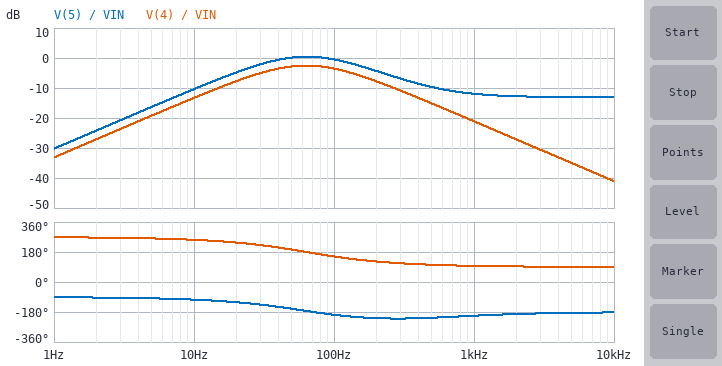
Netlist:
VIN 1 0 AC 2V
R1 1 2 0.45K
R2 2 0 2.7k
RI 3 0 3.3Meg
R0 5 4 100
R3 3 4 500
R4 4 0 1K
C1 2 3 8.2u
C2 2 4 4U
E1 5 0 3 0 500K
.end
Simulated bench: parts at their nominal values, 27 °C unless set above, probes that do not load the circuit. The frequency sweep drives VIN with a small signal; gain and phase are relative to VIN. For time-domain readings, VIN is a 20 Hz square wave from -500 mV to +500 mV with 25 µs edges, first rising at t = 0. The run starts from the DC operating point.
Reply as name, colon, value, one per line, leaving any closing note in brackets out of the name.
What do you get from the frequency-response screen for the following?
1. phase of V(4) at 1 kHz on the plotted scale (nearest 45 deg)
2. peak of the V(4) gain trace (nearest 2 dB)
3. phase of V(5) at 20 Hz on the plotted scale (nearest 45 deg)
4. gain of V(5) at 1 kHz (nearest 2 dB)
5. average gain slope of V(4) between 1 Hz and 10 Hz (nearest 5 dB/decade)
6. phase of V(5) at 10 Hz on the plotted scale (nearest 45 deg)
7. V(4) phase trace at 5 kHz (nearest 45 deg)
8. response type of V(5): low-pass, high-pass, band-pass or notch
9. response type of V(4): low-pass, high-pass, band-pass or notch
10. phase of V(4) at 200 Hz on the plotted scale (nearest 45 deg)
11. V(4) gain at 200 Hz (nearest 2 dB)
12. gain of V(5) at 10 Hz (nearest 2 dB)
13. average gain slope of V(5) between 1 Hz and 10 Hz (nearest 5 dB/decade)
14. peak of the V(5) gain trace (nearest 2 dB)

phase of V(4) at 1 kHz on the plotted scale: 90 deg
peak of the V(4) gain trace: -2 dB
phase of V(5) at 20 Hz on the plotted scale: -135 deg
gain of V(5) at 1 kHz: -12 dB
average gain slope of V(4) between 1 Hz and 10 Hz: 20 dB/decade
phase of V(5) at 10 Hz on the plotted scale: -90 deg
V(4) phase trace at 5 kHz: 90 deg
response type of V(5): low-pass, high-pass, band-pass or notch: band-pass
response type of V(4): low-pass, high-pass, band-pass or notch: band-pass
phase of V(4) at 200 Hz on the plotted scale: 135 deg
V(4) gain at 200 Hz: -8 dB
gain of V(5) at 10 Hz: -10 dB
average gain slope of V(5) between 1 Hz and 10 Hz: 20 dB/decade
peak of the V(5) gain trace: 0 dB
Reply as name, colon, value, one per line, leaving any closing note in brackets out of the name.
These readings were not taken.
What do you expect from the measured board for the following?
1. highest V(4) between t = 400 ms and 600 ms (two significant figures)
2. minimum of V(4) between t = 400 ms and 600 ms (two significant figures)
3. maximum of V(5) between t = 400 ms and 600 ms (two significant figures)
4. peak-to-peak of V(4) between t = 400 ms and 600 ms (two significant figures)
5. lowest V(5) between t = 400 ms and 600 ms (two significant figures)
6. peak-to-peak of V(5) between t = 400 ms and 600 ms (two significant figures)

highest V(4) between t = 400 ms and 600 ms: 540 mV
minimum of V(4) between t = 400 ms and 600 ms: -540 mV
maximum of V(5) between t = 400 ms and 600 ms: 760 mV
peak-to-peak of V(4) between t = 400 ms and 600 ms: 1.1 V
lowest V(5) between t = 400 ms and 600 ms: -760 mV
peak-to-peak of V(5) between t = 400 ms and 600 ms: 1.5 V
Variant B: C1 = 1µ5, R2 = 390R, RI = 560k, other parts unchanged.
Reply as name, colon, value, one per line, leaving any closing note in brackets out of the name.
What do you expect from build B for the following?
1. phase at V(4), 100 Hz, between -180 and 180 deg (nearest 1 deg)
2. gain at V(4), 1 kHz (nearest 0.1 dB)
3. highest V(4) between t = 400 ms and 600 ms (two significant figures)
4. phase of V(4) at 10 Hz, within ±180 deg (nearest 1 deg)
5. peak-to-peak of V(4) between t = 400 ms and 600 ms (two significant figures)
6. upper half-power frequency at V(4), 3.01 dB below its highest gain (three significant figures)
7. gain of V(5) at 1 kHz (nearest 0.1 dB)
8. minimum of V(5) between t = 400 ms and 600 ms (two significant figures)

phase at V(4), 100 Hz, between -180 and 180 deg: -134 deg
gain at V(4), 1 kHz: -21.1 dB
highest V(4) between t = 400 ms and 600 ms: 200 mV
phase of V(4) at 10 Hz, within ±180 deg: -94 deg
peak-to-peak of V(4) between t = 400 ms and 600 ms: 400 mV
upper half-power frequency at V(4), 3.01 dB below its highest gain: 394 Hz
gain of V(5) at 1 kHz: -11.2 dB
minimum of V(5) between t = 400 ms and 600 ms: -380 mV
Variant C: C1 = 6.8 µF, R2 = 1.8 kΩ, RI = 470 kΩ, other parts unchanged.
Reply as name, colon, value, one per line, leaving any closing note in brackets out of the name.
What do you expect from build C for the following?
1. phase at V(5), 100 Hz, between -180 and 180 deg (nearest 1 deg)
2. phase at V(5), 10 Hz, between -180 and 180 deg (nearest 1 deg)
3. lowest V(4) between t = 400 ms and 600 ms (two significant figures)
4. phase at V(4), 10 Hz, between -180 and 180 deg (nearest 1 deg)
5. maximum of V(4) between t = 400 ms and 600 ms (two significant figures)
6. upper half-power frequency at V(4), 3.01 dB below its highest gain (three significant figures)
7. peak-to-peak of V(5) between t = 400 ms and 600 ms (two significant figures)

phase at V(5), 100 Hz, between -180 and 180 deg: 169 deg
phase at V(5), 10 Hz, between -180 and 180 deg: -103 deg
lowest V(4) between t = 400 ms and 600 ms: -490 mV
phase at V(4), 10 Hz, between -180 and 180 deg: -104 deg
maximum of V(4) between t = 400 ms and 600 ms: 490 mV
upper half-power frequency at V(4), 3.01 dB below its highest gain: 159 Hz
peak-to-peak of V(5) between t = 400 ms and 600 ms: 1.4 V
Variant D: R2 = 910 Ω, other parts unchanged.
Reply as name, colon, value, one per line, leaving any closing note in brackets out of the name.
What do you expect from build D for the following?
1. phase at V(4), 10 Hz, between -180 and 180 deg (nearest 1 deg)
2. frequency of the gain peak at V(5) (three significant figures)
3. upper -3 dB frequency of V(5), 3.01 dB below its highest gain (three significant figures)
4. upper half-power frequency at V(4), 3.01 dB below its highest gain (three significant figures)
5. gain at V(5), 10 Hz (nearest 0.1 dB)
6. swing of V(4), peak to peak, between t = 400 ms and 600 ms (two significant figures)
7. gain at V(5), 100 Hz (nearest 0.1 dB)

phase at V(4), 10 Hz, between -180 and 180 deg: -103 deg
frequency of the gain peak at V(5): 72.4 Hz
upper -3 dB frequency of V(5), 3.01 dB below its highest gain: 158 Hz
upper half-power frequency at V(4), 3.01 dB below its highest gain: 152 Hz
gain at V(5), 10 Hz: -12.4 dB
swing of V(4), peak to peak, between t = 400 ms and 600 ms: 1.0 V
gain at V(5), 100 Hz: -0.2 dB
